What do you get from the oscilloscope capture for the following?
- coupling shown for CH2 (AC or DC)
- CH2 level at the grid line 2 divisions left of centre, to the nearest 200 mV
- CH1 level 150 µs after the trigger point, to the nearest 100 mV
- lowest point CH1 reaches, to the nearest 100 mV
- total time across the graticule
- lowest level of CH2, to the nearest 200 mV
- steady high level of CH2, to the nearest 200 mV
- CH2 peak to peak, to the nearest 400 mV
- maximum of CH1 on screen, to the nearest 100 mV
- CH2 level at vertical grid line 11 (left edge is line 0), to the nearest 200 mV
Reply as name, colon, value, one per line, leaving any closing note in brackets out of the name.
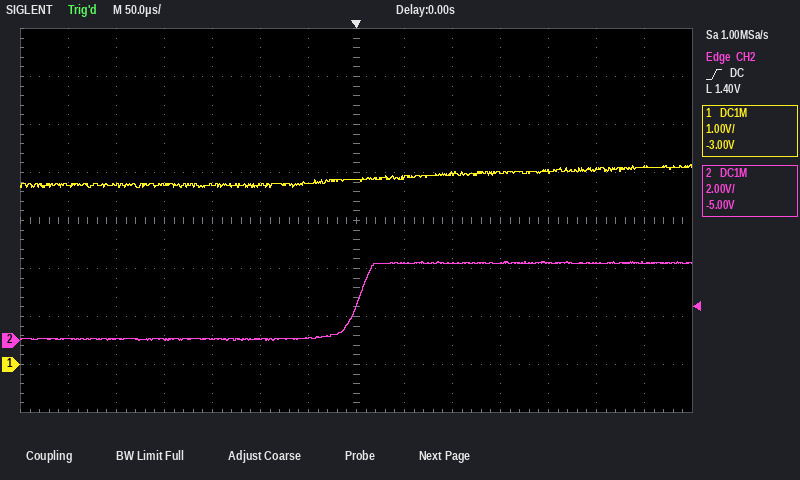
coupling shown for CH2: DC
CH2 level at the grid line 2 divisions left of centre, to the nearest 200 mV: 0.0 V
CH1 level 150 µs after the trigger point, to the nearest 100 mV: 4.0 V
lowest point CH1 reaches, to the nearest 100 mV: 3.7 V
total time across the graticule: 700 µs
lowest level of CH2, to the nearest 200 mV: 0.0 V
steady high level of CH2, to the nearest 200 mV: 3.2 V
CH2 peak to peak, to the nearest 400 mV: 3.2 V
maximum of CH1 on screen, to the nearest 100 mV: 4.2 V
CH2 level at vertical grid line 11 (left edge is line 0), to the nearest 200 mV: 3.2 V
